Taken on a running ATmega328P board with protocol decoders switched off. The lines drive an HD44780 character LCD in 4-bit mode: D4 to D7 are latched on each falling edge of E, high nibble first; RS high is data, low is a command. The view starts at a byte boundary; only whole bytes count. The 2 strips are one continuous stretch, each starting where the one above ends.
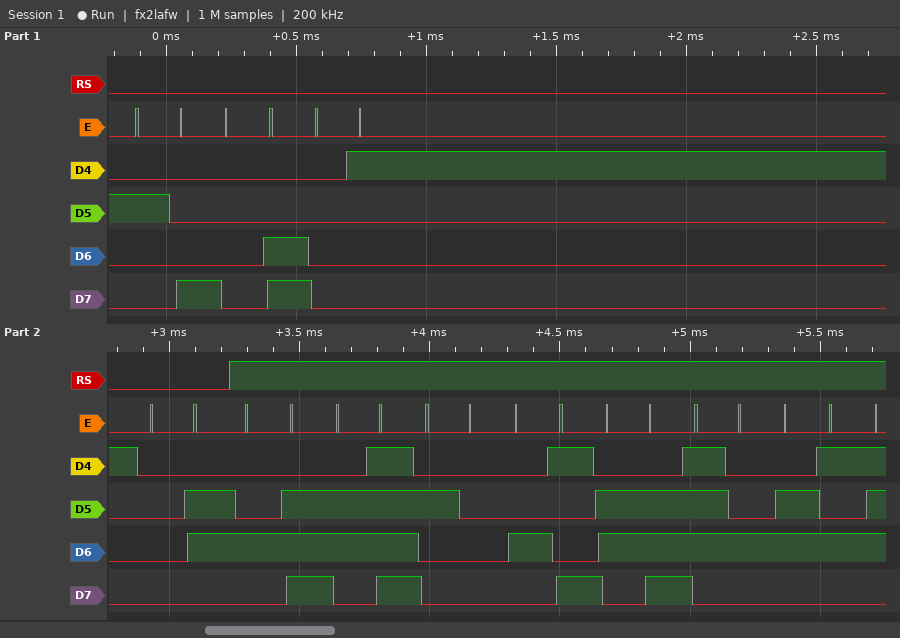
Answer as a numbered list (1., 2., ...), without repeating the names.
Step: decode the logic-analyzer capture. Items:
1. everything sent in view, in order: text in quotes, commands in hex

1. 0x28 0x0C 0x01 0x06 "No Inte"
